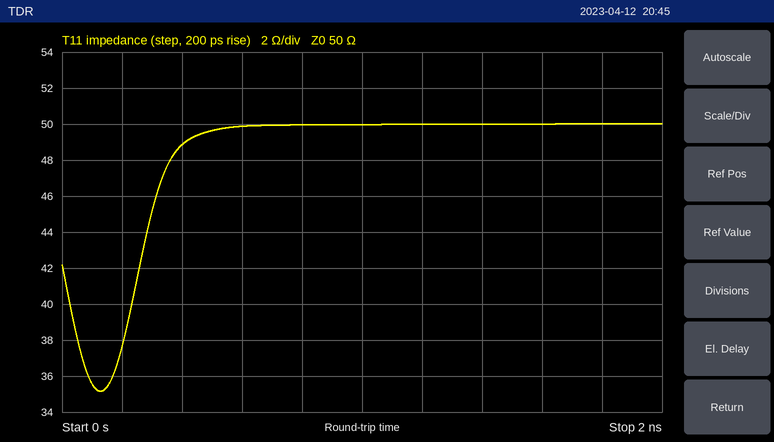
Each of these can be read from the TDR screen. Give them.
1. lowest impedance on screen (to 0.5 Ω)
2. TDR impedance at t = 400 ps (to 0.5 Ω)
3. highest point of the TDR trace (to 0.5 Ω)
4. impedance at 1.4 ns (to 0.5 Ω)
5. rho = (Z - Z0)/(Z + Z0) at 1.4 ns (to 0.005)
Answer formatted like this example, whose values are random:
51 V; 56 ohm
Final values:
35.0 Ω; 49.0 Ω; 50.0 Ω; 50.0 Ω; 0.000
